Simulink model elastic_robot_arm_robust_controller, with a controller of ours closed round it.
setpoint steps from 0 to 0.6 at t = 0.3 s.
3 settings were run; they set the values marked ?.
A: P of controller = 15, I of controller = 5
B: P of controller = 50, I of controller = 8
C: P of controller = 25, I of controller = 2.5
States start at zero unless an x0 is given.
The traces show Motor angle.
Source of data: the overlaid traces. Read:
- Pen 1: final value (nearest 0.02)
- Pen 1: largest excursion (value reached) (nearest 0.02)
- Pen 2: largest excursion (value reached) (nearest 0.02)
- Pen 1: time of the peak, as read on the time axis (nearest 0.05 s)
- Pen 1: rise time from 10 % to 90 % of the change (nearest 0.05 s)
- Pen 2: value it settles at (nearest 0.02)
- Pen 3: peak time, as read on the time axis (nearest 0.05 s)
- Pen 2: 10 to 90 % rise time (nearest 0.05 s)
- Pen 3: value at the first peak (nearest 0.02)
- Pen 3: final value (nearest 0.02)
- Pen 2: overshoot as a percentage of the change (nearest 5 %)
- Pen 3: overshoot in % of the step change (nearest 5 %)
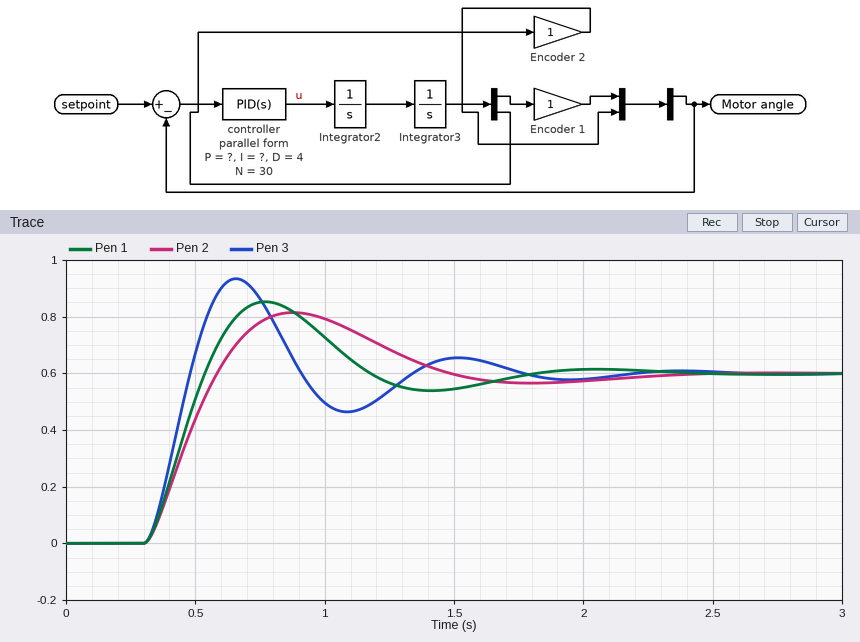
0.60
0.86
0.82
0.75 s
0.15 s
0.60
0.65 s
0.20 s
0.94
0.60
35 %
55 %
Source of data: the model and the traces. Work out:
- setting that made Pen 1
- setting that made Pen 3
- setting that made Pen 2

C
B
A
